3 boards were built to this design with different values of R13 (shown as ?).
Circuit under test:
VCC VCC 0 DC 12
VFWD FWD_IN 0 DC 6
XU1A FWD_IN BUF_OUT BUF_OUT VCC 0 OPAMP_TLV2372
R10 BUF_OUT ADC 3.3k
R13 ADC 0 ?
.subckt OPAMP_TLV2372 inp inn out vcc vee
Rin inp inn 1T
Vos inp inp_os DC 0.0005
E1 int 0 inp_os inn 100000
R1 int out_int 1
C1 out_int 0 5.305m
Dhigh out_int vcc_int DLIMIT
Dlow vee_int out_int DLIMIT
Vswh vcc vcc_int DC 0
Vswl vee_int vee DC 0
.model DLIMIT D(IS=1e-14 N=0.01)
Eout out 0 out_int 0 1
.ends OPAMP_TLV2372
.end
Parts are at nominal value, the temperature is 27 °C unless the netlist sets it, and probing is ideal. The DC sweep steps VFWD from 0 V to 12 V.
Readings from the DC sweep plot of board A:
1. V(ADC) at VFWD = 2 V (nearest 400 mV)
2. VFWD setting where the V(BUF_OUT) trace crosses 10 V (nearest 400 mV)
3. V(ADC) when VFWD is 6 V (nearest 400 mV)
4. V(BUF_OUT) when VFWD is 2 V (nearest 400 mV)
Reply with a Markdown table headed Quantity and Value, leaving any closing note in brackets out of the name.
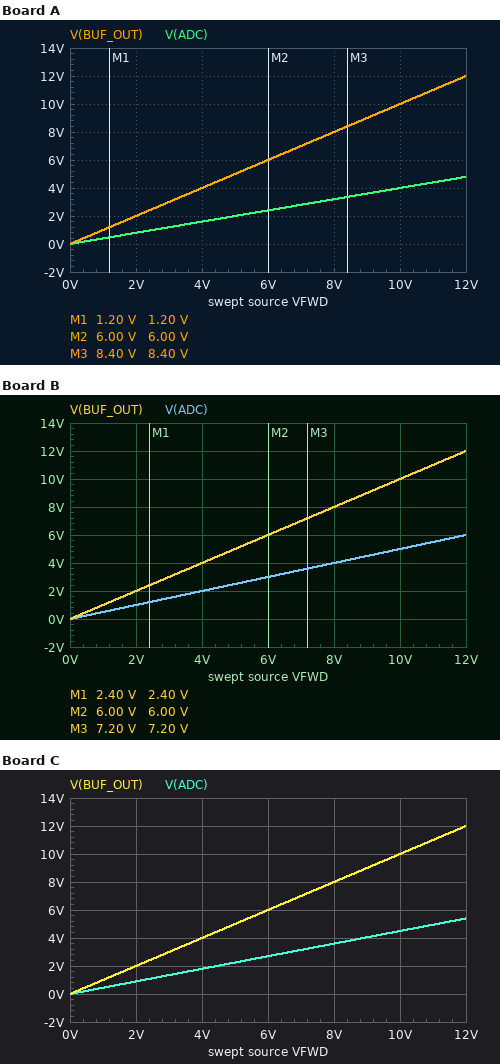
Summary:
| Quantity | Value |
|---|---|
| V(ADC) at VFWD = 2 V | 800 mV |
| VFWD setting where the V(BUF_OUT) trace crosses 10 V | 10.0 V |
| V(ADC) when VFWD is 6 V | 2.4 V |
| V(BUF_OUT) when VFWD is 2 V | 2.0 V |
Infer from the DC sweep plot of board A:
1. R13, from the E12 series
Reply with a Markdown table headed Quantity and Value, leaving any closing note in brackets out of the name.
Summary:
| Quantity | Value |
|---|---|
| R13, from the E12 series | 2.2 kΩ |
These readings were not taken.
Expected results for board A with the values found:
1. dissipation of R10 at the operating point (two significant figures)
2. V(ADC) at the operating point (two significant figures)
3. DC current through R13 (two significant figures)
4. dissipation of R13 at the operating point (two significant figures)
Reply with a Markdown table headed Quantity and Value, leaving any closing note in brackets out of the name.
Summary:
| Quantity | Value |
|---|---|
| dissipation of R10 at the operating point | 3.9 mW |
| V(ADC) at the operating point | 2.4 V |
| DC current through R13 | 1.1 mA |
| dissipation of R13 at the operating point | 2.6 mW |
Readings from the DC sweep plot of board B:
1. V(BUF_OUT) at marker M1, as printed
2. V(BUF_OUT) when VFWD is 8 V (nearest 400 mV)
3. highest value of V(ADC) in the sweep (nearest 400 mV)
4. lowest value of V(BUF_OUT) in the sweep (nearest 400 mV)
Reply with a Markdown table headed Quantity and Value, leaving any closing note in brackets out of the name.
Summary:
| Quantity | Value |
|---|---|
| V(BUF_OUT) at marker M1, as printed | 2.40 V |
| V(BUF_OUT) when VFWD is 8 V | 8.0 V |
| highest value of V(ADC) in the sweep | 6.0 V |
| lowest value of V(BUF_OUT) in the sweep | 0 V |
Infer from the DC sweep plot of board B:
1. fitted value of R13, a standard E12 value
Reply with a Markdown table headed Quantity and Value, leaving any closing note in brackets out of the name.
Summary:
| Quantity | Value |
|---|---|
| fitted value of R13, a standard E12 value | 3.3 kΩ |
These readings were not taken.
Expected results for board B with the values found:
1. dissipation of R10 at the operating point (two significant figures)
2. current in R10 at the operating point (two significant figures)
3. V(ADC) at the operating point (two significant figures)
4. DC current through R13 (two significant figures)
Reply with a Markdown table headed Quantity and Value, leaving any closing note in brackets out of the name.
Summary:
| Quantity | Value |
|---|---|
| dissipation of R10 at the operating point | 2.7 mW |
| current in R10 at the operating point | 910 µA |
| V(ADC) at the operating point | 3.0 V |
| DC current through R13 | 910 µA |
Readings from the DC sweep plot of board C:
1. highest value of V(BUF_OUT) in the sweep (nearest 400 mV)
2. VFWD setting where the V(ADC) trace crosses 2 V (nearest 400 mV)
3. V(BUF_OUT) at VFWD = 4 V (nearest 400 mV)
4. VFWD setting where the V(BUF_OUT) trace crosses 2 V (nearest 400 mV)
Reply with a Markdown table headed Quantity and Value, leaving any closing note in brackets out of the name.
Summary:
| Quantity | Value |
|---|---|
| highest value of V(BUF_OUT) in the sweep | 12.0 V |
| VFWD setting where the V(ADC) trace crosses 2 V | 4.4 V |
| V(BUF_OUT) at VFWD = 4 V | 4.0 V |
| VFWD setting where the V(BUF_OUT) trace crosses 2 V | 2.0 V |
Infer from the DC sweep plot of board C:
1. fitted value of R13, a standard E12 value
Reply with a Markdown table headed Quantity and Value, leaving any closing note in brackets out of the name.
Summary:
| Quantity | Value |
|---|---|
| fitted value of R13, a standard E12 value | 2.7 kΩ |
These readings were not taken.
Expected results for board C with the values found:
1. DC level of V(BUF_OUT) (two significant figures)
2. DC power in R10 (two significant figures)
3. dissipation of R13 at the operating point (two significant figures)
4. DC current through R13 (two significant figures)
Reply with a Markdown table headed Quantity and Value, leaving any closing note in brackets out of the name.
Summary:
| Quantity | Value |
|---|---|
| DC level of V(BUF_OUT) | 6.0 V |
| DC power in R10 | 3.3 mW |
| dissipation of R13 at the operating point | 2.7 mW |
| DC current through R13 | 1.0 mA |
